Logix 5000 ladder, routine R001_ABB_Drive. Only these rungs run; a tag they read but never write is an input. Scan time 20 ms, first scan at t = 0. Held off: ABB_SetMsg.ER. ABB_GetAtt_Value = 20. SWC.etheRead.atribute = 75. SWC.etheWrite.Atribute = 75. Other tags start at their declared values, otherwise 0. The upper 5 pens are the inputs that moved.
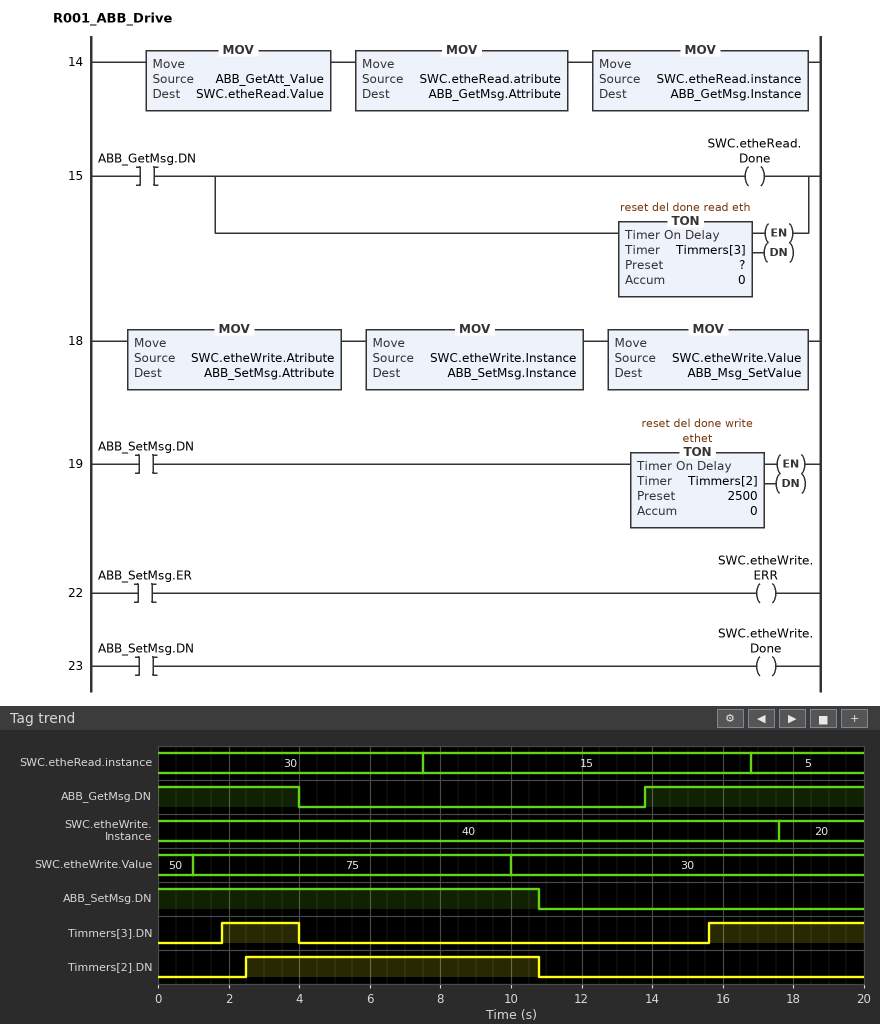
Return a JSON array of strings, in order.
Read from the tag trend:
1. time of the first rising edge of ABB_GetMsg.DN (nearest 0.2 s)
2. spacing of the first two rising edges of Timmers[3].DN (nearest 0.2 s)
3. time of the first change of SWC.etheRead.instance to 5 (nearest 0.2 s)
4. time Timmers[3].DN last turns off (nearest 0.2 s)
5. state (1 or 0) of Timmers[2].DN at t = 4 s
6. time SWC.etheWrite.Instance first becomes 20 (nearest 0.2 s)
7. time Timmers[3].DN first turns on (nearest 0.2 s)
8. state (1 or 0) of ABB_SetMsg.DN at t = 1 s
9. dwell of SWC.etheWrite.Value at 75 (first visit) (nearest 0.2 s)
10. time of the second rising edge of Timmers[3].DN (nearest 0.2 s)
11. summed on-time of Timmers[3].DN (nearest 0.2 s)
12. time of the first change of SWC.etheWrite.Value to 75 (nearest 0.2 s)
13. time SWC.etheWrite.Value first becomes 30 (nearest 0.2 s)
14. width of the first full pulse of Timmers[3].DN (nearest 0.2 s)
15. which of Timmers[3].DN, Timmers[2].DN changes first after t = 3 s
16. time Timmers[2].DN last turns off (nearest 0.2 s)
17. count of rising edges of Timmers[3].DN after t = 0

["13.8 s", "13.8 s", "16.8 s", "4.0 s", "1", "17.6 s", "1.8 s", "1", "9.0 s", "15.6 s", "6.6 s", "1.0 s", "10.0 s", "2.2 s", "Timmers[3].DN", "10.8 s", "2"]
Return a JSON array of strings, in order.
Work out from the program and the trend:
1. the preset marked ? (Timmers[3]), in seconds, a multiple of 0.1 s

["1.8 s"]
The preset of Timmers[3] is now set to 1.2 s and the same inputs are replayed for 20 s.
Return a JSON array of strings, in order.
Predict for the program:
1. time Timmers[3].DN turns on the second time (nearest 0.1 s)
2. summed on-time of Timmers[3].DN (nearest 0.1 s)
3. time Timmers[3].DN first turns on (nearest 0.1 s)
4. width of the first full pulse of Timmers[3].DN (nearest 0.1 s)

["15.0 s", "7.8 s", "1.2 s", "2.8 s"]
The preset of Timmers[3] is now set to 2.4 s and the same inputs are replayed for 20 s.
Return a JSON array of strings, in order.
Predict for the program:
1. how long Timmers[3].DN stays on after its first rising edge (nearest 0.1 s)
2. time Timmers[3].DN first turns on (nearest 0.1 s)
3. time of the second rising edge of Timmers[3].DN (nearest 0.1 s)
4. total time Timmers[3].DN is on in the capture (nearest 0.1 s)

["1.6 s", "2.4 s", "16.2 s", "5.4 s"]
